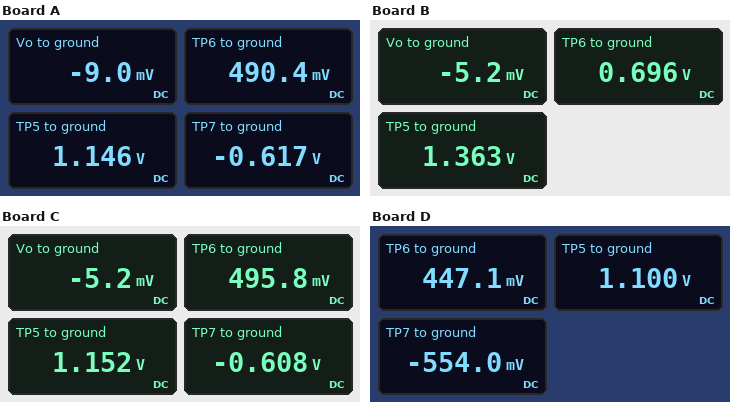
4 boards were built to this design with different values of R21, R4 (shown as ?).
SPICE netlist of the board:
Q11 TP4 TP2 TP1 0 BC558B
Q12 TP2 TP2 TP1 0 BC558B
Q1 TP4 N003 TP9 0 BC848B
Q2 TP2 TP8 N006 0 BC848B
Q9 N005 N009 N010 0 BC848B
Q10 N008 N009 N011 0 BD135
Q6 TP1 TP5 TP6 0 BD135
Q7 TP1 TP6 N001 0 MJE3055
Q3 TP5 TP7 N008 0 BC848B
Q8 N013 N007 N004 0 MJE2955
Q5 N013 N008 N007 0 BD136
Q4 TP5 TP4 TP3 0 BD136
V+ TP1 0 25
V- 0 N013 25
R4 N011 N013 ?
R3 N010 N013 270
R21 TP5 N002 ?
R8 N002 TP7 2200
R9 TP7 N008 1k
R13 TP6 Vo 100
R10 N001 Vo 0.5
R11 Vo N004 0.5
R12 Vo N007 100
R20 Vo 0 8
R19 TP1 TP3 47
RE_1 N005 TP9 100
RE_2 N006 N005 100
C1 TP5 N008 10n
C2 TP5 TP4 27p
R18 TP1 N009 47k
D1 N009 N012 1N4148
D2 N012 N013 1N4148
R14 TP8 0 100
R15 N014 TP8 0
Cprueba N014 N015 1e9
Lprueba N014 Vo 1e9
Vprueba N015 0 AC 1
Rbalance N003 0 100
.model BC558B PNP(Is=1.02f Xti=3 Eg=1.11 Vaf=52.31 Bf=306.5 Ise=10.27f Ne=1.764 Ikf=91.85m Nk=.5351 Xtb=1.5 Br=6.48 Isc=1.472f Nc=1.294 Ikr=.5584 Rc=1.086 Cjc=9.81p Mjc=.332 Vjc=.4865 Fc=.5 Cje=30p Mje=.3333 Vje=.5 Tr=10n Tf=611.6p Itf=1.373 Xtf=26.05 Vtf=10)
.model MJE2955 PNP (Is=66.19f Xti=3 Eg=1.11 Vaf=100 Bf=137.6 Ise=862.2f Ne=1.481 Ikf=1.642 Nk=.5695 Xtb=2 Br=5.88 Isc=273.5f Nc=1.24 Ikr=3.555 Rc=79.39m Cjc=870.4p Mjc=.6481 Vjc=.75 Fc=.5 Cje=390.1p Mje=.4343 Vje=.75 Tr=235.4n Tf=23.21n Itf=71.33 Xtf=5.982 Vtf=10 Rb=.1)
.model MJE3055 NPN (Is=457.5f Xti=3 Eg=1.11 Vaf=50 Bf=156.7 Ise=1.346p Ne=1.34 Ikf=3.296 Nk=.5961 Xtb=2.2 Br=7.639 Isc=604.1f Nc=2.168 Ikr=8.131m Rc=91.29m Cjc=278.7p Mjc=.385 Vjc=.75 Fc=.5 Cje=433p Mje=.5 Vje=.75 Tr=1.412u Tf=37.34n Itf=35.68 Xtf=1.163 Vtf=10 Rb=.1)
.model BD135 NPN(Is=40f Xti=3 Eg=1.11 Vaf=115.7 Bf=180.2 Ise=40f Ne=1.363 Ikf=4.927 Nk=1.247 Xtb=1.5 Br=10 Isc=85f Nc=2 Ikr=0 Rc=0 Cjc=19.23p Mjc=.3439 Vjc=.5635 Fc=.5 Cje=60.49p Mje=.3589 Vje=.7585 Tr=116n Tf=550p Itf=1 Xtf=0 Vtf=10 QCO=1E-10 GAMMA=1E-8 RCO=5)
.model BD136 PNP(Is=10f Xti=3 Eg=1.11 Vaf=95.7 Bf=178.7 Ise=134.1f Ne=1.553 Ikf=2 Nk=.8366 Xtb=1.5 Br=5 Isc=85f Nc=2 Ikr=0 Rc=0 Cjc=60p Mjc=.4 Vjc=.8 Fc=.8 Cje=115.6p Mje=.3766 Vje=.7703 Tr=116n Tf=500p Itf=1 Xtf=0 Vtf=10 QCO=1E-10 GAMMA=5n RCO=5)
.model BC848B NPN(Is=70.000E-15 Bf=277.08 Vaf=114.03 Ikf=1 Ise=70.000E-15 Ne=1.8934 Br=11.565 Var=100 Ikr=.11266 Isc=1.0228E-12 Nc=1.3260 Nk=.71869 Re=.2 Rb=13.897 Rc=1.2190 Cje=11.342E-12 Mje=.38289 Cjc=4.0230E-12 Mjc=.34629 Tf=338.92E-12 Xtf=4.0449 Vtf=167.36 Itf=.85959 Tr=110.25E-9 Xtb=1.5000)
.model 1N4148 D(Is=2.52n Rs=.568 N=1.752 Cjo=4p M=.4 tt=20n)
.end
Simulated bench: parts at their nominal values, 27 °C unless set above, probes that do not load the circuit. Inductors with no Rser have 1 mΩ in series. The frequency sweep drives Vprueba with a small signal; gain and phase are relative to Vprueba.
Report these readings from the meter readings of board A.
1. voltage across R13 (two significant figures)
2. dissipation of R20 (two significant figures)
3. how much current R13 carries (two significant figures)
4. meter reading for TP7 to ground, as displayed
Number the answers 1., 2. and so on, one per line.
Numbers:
1. 500 mV
2. 10 µW
3. 5.0 mA
4. -0.617 V
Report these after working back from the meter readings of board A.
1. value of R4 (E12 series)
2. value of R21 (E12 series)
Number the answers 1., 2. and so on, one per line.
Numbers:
1. 39 Ω
2. 270 Ω
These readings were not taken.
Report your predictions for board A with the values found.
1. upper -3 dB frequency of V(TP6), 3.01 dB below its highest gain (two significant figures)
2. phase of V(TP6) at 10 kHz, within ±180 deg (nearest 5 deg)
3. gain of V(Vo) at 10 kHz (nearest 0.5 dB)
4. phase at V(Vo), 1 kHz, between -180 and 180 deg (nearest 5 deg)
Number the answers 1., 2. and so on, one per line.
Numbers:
1. 3.7 kHz
2. 110 deg
3. 57.0 dB
4. 165 deg
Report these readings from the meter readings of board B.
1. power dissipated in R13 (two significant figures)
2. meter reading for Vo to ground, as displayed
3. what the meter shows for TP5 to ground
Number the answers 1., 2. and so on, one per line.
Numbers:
1. 4.9 mW
2. -5.2 mV
3. 1.363 V
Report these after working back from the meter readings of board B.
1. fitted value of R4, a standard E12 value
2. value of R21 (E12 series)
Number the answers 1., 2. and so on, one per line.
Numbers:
1. 68 Ω
2. 1 kΩ
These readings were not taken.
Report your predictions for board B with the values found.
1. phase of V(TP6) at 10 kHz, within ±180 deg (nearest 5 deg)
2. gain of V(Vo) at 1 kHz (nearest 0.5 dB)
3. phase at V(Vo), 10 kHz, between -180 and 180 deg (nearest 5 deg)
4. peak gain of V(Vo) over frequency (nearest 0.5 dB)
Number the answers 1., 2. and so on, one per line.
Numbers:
1. 100 deg
2. 84.0 dB
3. 100 deg
4. 85.5 dB
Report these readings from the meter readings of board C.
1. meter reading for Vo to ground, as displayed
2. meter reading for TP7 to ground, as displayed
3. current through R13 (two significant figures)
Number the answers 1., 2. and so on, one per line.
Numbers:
1. -5.2 mV
2. -0.608 V
3. 5.0 mA
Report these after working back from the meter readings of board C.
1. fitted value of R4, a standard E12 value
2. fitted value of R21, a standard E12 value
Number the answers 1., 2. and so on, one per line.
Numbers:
1. 68 Ω
2. 390 Ω
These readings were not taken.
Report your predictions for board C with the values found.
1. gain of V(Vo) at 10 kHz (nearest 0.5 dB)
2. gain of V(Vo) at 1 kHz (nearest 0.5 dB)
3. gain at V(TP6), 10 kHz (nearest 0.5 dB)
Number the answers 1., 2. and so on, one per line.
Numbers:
1. 55.5 dB
2. 66.0 dB
3. 68.5 dB
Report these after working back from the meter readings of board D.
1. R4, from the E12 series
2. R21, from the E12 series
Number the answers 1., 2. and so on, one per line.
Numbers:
1. 82 Ω
2. 270 Ω
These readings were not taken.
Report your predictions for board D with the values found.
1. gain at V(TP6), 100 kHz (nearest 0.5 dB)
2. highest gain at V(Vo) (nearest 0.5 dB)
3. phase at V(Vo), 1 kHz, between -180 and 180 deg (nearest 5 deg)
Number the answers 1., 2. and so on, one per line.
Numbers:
1. 49.0 dB
2. 63.0 dB
3. 160 deg
